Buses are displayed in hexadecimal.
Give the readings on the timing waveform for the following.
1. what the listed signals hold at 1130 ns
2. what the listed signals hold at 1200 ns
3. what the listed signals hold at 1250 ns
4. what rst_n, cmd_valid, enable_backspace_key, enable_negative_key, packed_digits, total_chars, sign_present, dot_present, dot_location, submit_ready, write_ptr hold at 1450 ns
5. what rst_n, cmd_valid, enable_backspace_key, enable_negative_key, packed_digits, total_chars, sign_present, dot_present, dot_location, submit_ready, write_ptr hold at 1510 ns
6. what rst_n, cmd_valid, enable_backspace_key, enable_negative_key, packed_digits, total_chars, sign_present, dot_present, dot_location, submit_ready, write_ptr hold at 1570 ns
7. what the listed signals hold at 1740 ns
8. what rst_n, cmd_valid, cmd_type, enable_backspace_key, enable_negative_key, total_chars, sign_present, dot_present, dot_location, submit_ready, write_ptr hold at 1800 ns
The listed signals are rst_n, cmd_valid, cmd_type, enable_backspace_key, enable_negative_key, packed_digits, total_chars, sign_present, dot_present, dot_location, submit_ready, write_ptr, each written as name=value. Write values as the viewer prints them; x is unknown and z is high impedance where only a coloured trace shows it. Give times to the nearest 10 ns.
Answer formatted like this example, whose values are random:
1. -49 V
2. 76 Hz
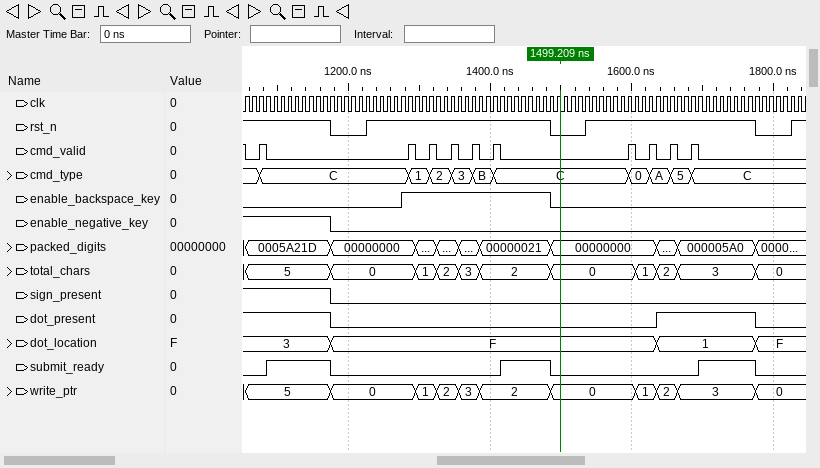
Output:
1. rst_n=1, cmd_valid=0, cmd_type=C, enable_backspace_key=0, enable_negative_key=1, packed_digits=0005A21D, total_chars=5, sign_present=1, dot_present=1, dot_location=3, submit_ready=1, write_ptr=5
2. rst_n=0, cmd_valid=0, cmd_type=C, enable_backspace_key=0, enable_negative_key=0, packed_digits=00000000, total_chars=0, sign_present=0, dot_present=0, dot_location=F, submit_ready=0, write_ptr=0
3. rst_n=1, cmd_valid=0, cmd_type=C, enable_backspace_key=0, enable_negative_key=0, packed_digits=00000000, total_chars=0, sign_present=0, dot_present=0, dot_location=F, submit_ready=0, write_ptr=0
4. rst_n=1, cmd_valid=0, enable_backspace_key=1, enable_negative_key=0, packed_digits=00000021, total_chars=2, sign_present=0, dot_present=0, dot_location=F, submit_ready=1, write_ptr=2
5. rst_n=0, cmd_valid=0, enable_backspace_key=0, enable_negative_key=0, packed_digits=00000000, total_chars=0, sign_present=0, dot_present=0, dot_location=F, submit_ready=0, write_ptr=0
6. rst_n=1, cmd_valid=0, enable_backspace_key=0, enable_negative_key=0, packed_digits=00000000, total_chars=0, sign_present=0, dot_present=0, dot_location=F, submit_ready=0, write_ptr=0
7. rst_n=1, cmd_valid=0, cmd_type=C, enable_backspace_key=0, enable_negative_key=0, packed_digits=000005A0, total_chars=3, sign_present=0, dot_present=1, dot_location=1, submit_ready=1, write_ptr=3
8. rst_n=0, cmd_valid=0, cmd_type=C, enable_backspace_key=0, enable_negative_key=0, total_chars=0, sign_present=0, dot_present=0, dot_location=F, submit_ready=0, write_ptr=0
